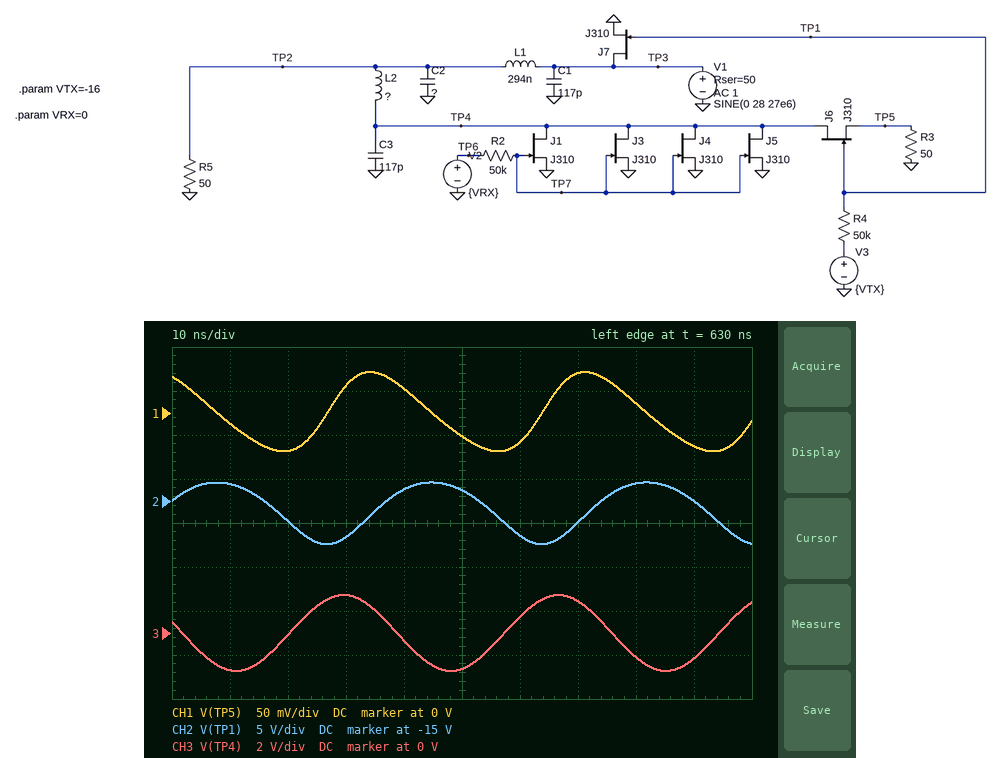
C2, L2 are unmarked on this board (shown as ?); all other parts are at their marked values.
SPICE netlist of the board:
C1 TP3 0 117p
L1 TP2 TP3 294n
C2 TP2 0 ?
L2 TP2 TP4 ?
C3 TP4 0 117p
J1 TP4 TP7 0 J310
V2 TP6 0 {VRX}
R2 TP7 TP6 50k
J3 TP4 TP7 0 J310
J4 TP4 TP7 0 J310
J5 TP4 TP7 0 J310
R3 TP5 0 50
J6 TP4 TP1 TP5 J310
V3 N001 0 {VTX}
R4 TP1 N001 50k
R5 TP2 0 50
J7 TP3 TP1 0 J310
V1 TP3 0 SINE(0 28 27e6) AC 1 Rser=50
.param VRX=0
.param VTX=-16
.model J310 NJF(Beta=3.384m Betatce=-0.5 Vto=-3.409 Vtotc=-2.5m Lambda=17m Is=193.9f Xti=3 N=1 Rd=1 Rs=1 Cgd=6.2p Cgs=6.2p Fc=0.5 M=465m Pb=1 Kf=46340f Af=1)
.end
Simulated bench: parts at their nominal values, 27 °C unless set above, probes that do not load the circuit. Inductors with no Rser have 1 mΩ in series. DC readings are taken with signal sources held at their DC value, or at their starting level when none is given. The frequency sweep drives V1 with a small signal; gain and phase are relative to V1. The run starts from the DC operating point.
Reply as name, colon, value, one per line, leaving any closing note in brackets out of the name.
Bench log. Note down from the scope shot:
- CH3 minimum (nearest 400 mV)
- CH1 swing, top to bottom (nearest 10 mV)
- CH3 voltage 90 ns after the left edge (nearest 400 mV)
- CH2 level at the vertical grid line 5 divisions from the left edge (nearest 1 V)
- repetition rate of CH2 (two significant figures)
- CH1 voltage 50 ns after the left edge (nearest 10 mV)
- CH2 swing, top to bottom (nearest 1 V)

CH3 minimum: -1.6 V
CH1 swing, top to bottom: 90 mV
CH3 voltage 90 ns after the left edge: -1.2 V
CH2 level at the vertical grid line 5 divisions from the left edge: -14 V
repetition rate of CH2: 27 MHz
CH1 voltage 50 ns after the left edge: -30 mV
CH2 swing, top to bottom: 7 V
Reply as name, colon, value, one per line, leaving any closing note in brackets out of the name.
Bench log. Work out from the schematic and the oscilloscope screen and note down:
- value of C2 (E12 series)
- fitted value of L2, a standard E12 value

value of C2: 220 pF
fitted value of L2, a standard E12 value: 560 nH
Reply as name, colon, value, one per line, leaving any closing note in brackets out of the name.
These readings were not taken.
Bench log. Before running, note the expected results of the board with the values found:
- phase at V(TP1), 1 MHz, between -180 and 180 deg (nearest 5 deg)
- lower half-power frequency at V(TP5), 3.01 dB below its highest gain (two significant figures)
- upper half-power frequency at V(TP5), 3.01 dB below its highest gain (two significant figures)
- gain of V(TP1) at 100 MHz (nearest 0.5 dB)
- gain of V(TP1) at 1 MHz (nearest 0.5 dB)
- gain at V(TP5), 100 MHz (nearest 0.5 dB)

phase at V(TP1), 1 MHz, between -180 and 180 deg: 35 deg
lower half-power frequency at V(TP5), 3.01 dB below its highest gain: 32 MHz
upper half-power frequency at V(TP5), 3.01 dB below its highest gain: 1.8 GHz
gain of V(TP1) at 100 MHz: -23.0 dB
gain of V(TP1) at 1 MHz: -23.0 dB
gain at V(TP5), 100 MHz: -49.5 dB
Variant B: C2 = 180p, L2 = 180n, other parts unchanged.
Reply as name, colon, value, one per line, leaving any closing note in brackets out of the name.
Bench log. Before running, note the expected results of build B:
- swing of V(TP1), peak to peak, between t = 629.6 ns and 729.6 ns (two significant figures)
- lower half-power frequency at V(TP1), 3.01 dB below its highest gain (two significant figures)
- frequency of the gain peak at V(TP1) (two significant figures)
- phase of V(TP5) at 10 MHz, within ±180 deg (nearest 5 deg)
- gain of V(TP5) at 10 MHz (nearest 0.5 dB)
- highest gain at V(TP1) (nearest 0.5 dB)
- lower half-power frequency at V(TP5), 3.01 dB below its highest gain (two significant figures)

swing of V(TP1), peak to peak, between t = 629.6 ns and 729.6 ns: 8.3 V
lower half-power frequency at V(TP1), 3.01 dB below its highest gain: 8.7 MHz
frequency of the gain peak at V(TP1): 20 MHz
phase of V(TP5) at 10 MHz, within ±180 deg: 110 deg
gain of V(TP5) at 10 MHz: -65.0 dB
highest gain at V(TP1): -16.0 dB
lower half-power frequency at V(TP5), 3.01 dB below its highest gain: 38 MHz
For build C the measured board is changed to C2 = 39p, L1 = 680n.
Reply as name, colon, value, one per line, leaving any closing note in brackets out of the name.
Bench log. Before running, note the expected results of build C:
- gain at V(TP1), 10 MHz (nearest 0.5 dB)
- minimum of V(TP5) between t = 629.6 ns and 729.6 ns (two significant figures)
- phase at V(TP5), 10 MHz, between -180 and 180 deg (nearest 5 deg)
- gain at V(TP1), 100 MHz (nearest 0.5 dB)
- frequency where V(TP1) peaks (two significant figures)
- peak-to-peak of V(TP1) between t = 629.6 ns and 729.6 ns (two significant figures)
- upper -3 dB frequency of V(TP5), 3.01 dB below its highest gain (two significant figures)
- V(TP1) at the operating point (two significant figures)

gain at V(TP1), 10 MHz: -14.5 dB
minimum of V(TP5) between t = 629.6 ns and 729.6 ns: -73 mV
phase at V(TP5), 10 MHz, between -180 and 180 deg: 100 deg
gain at V(TP1), 100 MHz: -23.5 dB
frequency where V(TP1) peaks: 17 MHz
peak-to-peak of V(TP1) between t = 629.6 ns and 729.6 ns: 11 V
upper -3 dB frequency of V(TP5), 3.01 dB below its highest gain: 2.8 GHz
V(TP1) at the operating point: -16 V
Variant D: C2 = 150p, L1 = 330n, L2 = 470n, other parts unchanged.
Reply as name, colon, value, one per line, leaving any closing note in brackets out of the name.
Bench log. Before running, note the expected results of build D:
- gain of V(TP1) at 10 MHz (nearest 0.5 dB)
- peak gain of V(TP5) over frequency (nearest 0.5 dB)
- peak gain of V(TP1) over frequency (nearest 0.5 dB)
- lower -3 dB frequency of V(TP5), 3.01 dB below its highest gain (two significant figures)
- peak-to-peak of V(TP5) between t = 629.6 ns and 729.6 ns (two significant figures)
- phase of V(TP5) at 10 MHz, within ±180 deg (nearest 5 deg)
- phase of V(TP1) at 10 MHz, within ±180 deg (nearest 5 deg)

gain of V(TP1) at 10 MHz: -17.0 dB
peak gain of V(TP5) over frequency: -49.0 dB
peak gain of V(TP1) over frequency: -15.0 dB
lower -3 dB frequency of V(TP5), 3.01 dB below its highest gain: 34 MHz
peak-to-peak of V(TP5) between t = 629.6 ns and 729.6 ns: 99 mV
phase of V(TP5) at 10 MHz, within ±180 deg: 100 deg
phase of V(TP1) at 10 MHz, within ±180 deg: 10 deg
